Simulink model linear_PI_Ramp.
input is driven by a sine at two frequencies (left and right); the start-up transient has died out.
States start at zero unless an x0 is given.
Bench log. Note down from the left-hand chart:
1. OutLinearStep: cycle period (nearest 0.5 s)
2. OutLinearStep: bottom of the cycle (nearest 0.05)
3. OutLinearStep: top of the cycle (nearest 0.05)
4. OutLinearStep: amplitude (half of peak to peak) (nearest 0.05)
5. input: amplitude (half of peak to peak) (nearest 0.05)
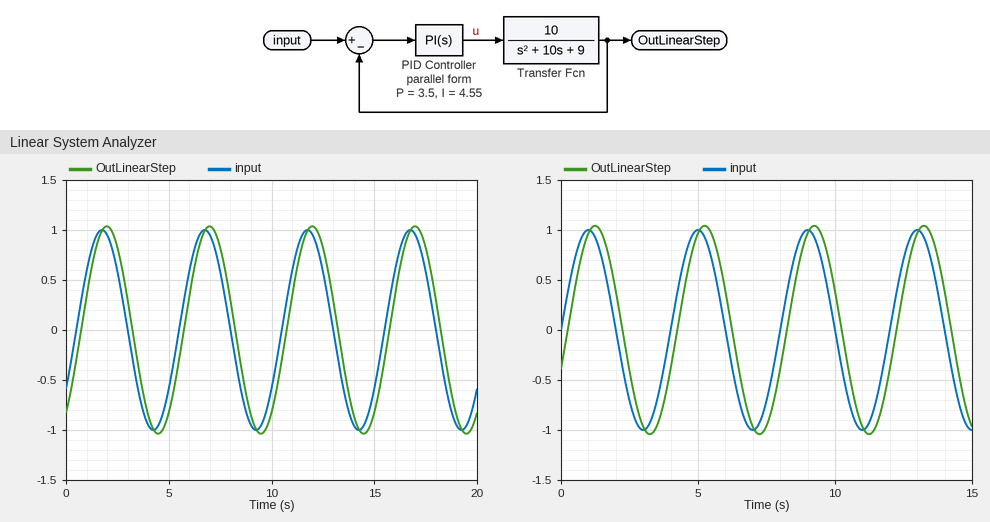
5.0 s
-1.05
1.05
1.05
1.00
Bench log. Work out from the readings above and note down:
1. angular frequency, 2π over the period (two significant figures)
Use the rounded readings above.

1.3 rad/s
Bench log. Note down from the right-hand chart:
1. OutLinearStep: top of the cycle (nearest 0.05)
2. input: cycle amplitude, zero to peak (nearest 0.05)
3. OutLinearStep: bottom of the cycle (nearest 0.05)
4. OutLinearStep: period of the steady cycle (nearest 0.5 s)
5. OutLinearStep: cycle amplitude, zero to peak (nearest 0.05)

1.05
1.00
-1.05
4.0 s
1.05
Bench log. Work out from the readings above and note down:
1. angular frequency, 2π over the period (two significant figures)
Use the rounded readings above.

1.6 rad/s
